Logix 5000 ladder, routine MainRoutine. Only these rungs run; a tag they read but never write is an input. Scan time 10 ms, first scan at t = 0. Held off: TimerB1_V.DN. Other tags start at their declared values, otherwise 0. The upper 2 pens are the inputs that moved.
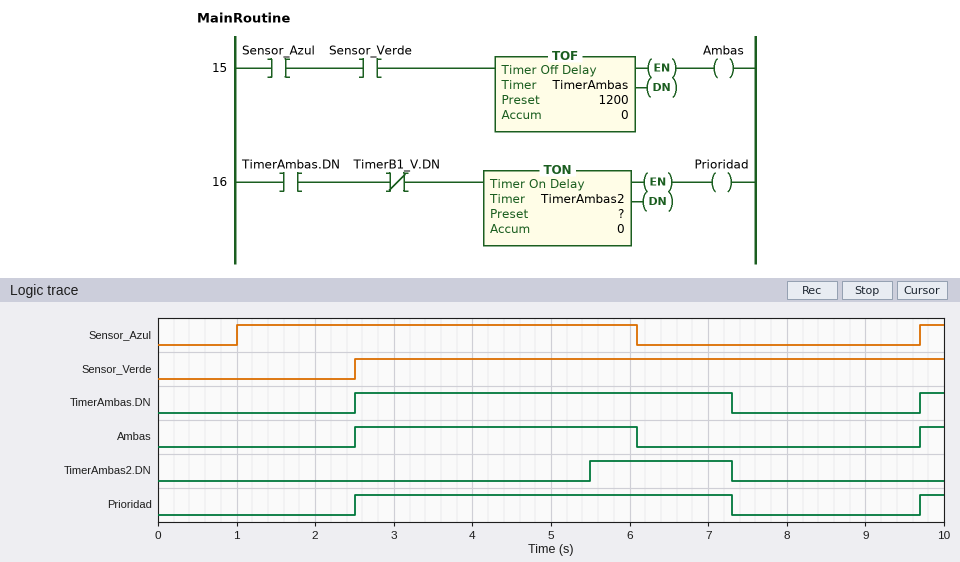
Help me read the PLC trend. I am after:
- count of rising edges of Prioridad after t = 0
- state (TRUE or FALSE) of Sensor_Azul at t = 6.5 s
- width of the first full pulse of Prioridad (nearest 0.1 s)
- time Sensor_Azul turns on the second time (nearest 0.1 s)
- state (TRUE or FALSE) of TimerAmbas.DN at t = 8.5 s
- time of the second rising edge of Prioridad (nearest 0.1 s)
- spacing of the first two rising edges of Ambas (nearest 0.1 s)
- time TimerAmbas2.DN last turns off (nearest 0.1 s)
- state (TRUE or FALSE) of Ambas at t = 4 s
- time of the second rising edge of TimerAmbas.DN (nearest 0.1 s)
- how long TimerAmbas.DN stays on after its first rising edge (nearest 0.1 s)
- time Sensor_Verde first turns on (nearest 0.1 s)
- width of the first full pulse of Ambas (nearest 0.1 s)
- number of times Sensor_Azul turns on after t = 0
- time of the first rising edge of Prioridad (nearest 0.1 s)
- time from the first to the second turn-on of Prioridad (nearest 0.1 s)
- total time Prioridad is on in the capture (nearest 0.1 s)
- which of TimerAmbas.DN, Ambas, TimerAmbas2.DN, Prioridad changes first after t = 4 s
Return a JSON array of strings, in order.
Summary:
["2", "FALSE", "4.8 s", "9.7 s", "FALSE", "9.7 s", "7.2 s", "7.3 s", "TRUE", "9.7 s", "4.8 s", "2.5 s", "3.6 s", "2", "2.5 s", "7.2 s", "5.1 s", "TimerAmbas2.DN"]
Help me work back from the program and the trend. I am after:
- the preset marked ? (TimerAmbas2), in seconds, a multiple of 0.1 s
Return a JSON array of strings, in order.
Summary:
["3.0 s"]
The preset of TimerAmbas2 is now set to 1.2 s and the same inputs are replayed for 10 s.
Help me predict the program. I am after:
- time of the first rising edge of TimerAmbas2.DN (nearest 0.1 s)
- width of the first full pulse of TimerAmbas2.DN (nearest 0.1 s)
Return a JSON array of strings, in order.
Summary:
["3.7 s", "3.6 s"]
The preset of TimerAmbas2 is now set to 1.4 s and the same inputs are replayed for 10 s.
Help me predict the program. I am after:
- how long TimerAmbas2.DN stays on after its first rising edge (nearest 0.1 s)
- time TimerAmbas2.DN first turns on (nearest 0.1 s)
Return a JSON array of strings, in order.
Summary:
["3.4 s", "3.9 s"]
